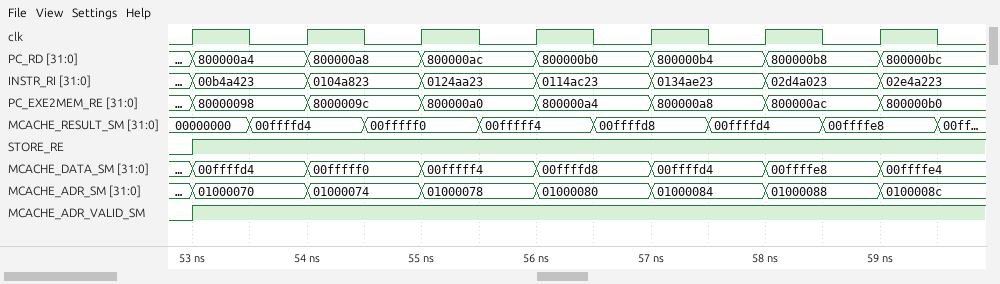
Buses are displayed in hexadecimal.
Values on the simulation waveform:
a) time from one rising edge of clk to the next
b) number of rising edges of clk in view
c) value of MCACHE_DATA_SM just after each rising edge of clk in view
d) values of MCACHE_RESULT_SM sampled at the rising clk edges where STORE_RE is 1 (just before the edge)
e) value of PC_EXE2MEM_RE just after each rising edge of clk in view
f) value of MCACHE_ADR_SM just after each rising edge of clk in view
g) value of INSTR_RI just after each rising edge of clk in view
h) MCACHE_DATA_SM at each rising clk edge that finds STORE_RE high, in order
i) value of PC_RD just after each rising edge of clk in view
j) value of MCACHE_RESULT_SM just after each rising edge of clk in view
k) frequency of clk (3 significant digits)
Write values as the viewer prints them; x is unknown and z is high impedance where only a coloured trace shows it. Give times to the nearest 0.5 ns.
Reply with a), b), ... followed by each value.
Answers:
a) 1 ns
b) 7
c) 00ffffd4, 00fffff0, 00fffff4, 00ffffd8, 00ffffd4, 00ffffe8, 00ffffe4
d) 00ffffd4, 00fffff0, 00fffff4, 00ffffd8, 00ffffd4, 00ffffe8
e) 80000098, 8000009c, 800000a0, 800000a4, 800000a8, 800000ac, 800000b0
f) 01000070, 01000074, 01000078, 01000080, 01000084, 01000088, 0100008c
g) 00b4a423, 0104a823, 0124aa23, 0114ac23, 0134ae23, 02d4a023, 02e4a223
h) 00ffffd4, 00fffff0, 00fffff4, 00ffffd8, 00ffffd4, 00ffffe8
i) 800000a4, 800000a8, 800000ac, 800000b0, 800000b4, 800000b8, 800000bc
j) 00000000, 00ffffd4, 00fffff0, 00fffff4, 00ffffd8, 00ffffd4, 00ffffe8
k) 1.00 GHz
